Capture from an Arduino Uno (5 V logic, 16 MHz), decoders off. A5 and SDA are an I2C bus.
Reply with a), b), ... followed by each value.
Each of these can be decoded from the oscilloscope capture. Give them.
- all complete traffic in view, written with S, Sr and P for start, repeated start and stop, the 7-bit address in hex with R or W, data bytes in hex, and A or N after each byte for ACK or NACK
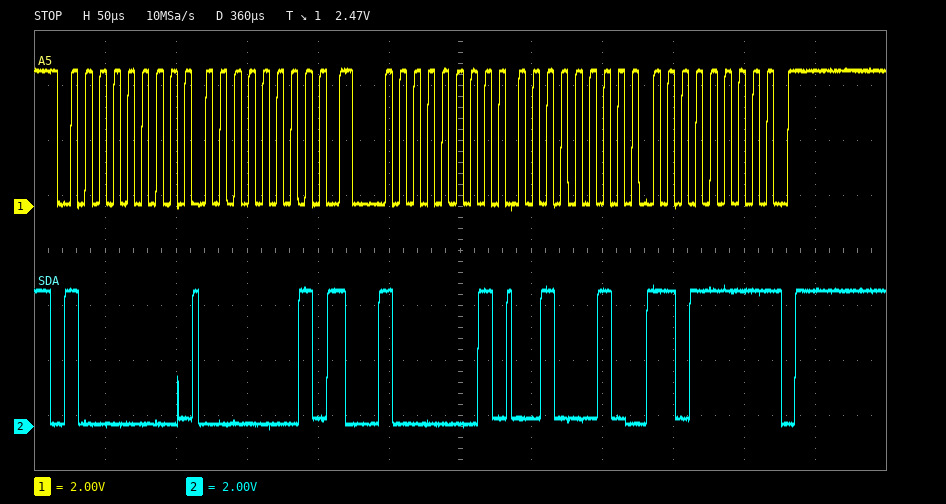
a) S 40W A 01 A Sr 40R A 22 A DF N P
